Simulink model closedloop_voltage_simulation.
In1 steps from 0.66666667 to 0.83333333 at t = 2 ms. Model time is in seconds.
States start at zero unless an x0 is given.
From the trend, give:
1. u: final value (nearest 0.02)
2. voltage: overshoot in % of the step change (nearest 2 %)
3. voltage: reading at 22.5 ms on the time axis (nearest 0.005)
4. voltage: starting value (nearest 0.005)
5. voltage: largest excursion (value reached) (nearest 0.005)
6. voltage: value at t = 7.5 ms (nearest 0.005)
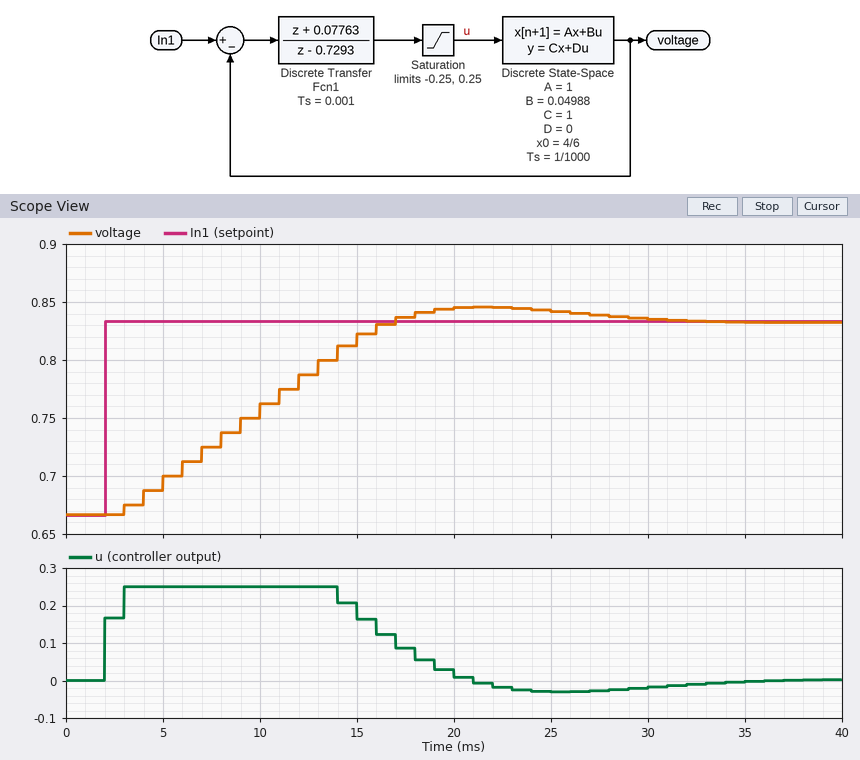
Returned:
0.00
8 %
0.845
0.665
0.845
0.725
